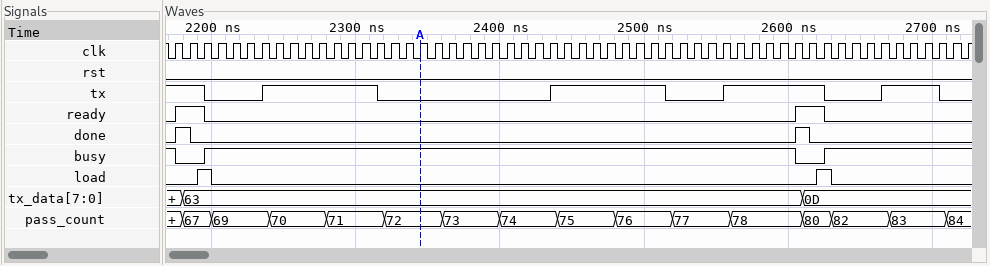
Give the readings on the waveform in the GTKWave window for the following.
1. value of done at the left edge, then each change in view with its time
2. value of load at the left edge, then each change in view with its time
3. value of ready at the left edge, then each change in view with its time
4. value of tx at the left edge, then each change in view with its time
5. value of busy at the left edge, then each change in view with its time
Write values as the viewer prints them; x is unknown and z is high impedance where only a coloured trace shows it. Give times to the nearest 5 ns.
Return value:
0, 1 at 2175 ns, 0 at 2185 ns, 1 at 2605 ns, 0 at 2615 ns
0, 1 at 2190 ns, 0 at 2200 ns, 1 at 2620 ns, 0 at 2630 ns
0, 1 at 2175 ns, 0 at 2195 ns, 1 at 2605 ns, 0 at 2625 ns
1, 0 at 2195 ns, 1 at 2235 ns, 0 at 2315 ns, 1 at 2435 ns, 0 at 2515 ns, 1 at 2555 ns, 0 at 2625 ns, 1 at 2665 ns, 0 at 2705 ns
1, 0 at 2175 ns, 1 at 2195 ns, 0 at 2605 ns, 1 at 2625 ns
